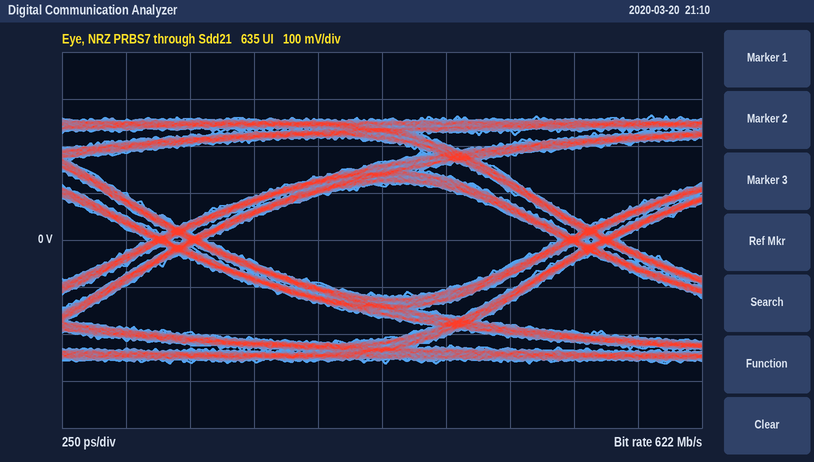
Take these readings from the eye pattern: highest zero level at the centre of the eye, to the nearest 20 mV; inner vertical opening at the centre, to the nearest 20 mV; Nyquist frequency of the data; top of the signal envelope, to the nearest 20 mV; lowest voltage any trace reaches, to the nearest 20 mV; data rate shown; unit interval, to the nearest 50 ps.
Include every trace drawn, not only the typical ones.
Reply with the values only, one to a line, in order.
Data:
-120 mV
240 mV
311 MHz
260 mV
-260 mV
622 Mb/s
1.60 ns
